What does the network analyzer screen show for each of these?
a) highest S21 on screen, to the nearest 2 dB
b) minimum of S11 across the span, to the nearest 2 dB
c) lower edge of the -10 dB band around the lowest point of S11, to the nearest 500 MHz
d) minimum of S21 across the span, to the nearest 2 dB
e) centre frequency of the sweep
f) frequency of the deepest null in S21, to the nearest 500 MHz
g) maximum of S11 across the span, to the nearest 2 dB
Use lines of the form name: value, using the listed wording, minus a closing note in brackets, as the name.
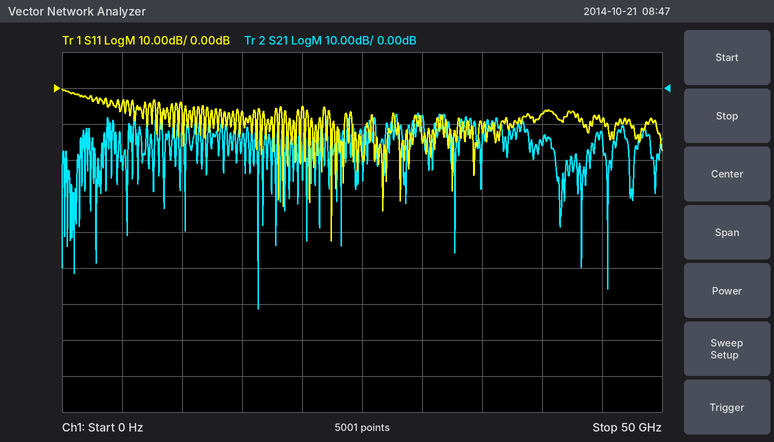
highest S21 on screen, to the nearest 2 dB: -6 dB
minimum of S11 across the span, to the nearest 2 dB: -42 dB
lower edge of the -10 dB band around the lowest point of S11, to the nearest 500 MHz: 22.5 GHz
minimum of S21 across the span, to the nearest 2 dB: -62 dB
centre frequency of the sweep: 25 GHz
frequency of the deepest null in S21, to the nearest 500 MHz: 16.5 GHz
maximum of S11 across the span, to the nearest 2 dB: 0 dB
